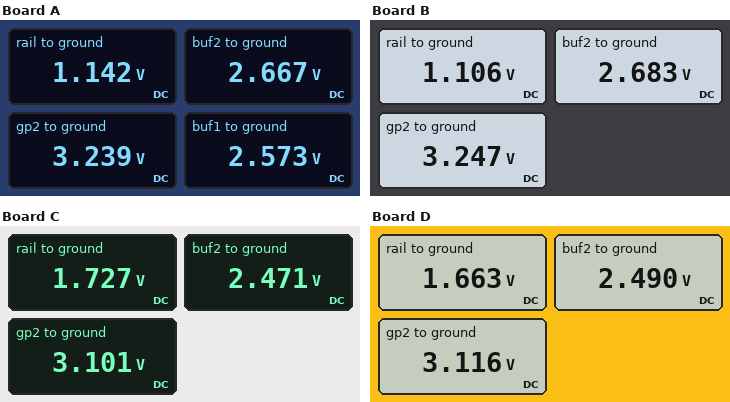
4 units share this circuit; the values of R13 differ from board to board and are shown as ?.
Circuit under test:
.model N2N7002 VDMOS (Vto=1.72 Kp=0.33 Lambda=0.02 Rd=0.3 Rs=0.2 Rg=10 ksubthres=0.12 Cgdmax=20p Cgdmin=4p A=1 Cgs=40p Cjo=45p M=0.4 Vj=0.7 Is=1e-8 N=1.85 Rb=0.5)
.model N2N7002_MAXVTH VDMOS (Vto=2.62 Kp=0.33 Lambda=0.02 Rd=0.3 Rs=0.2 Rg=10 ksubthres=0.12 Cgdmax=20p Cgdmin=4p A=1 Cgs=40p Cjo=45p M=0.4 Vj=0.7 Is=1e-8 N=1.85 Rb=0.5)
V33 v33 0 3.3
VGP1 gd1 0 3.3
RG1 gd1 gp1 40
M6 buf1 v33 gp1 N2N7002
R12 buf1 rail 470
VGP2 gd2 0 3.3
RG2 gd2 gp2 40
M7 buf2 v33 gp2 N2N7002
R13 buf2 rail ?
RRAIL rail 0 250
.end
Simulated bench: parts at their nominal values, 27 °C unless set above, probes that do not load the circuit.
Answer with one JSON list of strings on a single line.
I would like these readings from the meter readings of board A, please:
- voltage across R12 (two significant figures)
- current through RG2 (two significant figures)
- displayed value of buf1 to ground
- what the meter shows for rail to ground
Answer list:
["1.4 V", "1.5 mA", "2.573 V", "1.142 V"]
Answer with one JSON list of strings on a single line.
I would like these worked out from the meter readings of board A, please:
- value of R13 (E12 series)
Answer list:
["1 kΩ"]
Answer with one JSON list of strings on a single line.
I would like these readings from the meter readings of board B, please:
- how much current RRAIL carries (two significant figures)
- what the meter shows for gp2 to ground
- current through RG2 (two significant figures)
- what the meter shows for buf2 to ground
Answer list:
["4.4 mA", "3.247 V", "1.3 mA", "2.683 V"]
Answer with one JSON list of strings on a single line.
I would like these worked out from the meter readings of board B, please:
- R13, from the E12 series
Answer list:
["1.2 kΩ"]
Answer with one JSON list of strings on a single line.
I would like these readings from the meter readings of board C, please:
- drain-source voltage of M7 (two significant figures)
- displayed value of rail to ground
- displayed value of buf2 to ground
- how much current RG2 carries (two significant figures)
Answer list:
["-630 mV", "1.727 V", "2.471 V", "5.0 mA"]
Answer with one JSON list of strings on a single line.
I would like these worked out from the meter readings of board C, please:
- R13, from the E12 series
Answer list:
["150 Ω"]
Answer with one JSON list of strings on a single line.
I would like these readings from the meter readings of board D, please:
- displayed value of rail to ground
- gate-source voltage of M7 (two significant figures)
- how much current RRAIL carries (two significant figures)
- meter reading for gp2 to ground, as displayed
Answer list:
["1.663 V", "180 mV", "6.7 mA", "3.116 V"]
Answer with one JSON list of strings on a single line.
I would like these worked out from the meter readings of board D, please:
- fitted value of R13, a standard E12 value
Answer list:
["180 Ω"]
